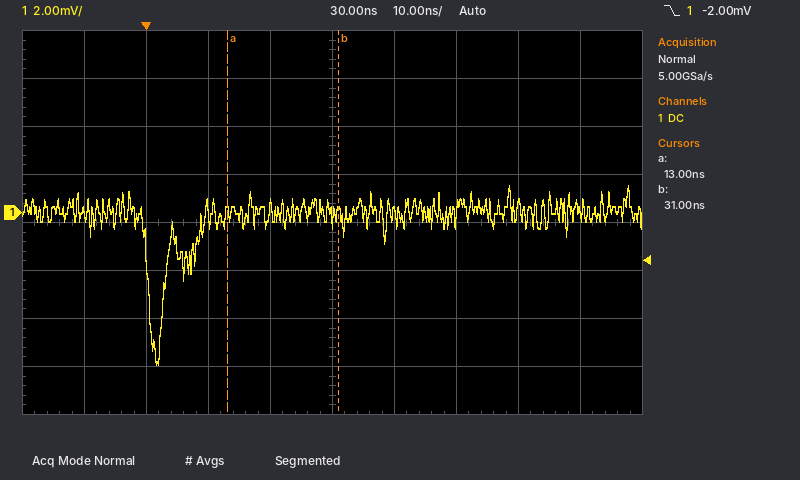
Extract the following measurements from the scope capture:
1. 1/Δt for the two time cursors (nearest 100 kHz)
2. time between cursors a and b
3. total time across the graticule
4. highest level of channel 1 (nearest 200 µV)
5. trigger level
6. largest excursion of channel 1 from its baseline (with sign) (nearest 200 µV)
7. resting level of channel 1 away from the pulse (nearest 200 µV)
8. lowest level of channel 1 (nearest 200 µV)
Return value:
55.6 MHz
18 ns
100 ns
1.2 mV
-2.00 mV
-6.4 mV
0.0 mV
-6.4 mV
